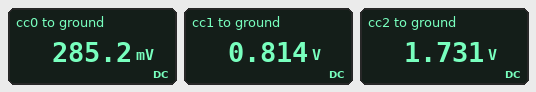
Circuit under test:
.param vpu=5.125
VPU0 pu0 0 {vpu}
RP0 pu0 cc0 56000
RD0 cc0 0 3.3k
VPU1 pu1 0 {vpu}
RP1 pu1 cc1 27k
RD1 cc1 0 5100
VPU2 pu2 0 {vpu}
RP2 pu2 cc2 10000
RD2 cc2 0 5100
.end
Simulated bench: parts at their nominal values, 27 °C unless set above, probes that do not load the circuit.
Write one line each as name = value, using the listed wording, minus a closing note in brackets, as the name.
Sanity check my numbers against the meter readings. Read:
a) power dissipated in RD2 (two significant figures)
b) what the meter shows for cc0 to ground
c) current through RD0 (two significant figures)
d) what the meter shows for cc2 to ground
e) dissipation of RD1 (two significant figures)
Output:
power dissipated in RD2 = 590 µW
what the meter shows for cc0 to ground = 285.2 mV
current through RD0 = 86 µA
what the meter shows for cc2 to ground = 1.731 V
dissipation of RD1 = 130 µW
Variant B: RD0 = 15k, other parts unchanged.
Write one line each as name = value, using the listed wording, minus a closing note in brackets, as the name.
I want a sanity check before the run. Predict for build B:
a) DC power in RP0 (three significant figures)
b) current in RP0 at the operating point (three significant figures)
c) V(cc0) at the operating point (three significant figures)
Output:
DC power in RP0 = 292 µW
current in RP0 at the operating point = 72.2 µA
V(cc0) at the operating point = 1.08 V
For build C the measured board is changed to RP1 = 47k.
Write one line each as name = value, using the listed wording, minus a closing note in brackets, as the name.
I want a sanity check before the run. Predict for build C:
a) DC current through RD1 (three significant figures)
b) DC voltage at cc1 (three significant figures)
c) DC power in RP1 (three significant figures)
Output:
DC current through RD1 = 98.4 µA
DC voltage at cc1 = 502 mV
DC power in RP1 = 455 µW
